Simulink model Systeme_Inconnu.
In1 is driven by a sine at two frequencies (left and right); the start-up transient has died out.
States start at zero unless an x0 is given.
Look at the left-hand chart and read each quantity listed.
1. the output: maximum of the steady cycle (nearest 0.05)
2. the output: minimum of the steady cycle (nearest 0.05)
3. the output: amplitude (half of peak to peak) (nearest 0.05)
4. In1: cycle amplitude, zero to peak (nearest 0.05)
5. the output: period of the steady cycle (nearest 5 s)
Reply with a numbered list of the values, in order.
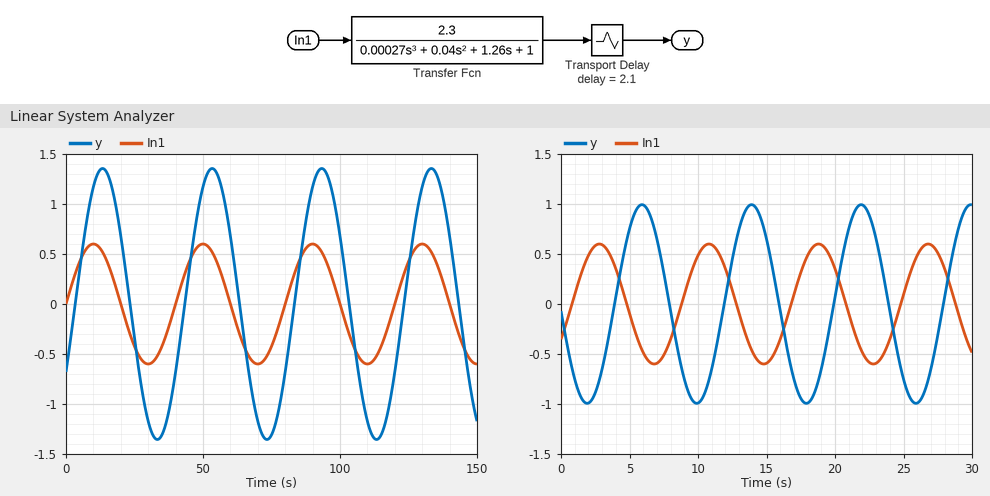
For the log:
1. 1.35
2. -1.35
3. 1.35
4. 0.60
5. 40 s
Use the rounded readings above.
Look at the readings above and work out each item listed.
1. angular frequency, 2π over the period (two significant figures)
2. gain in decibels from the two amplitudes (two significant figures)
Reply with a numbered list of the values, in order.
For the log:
1. 0.16 rad/s
2. 7.0 dB
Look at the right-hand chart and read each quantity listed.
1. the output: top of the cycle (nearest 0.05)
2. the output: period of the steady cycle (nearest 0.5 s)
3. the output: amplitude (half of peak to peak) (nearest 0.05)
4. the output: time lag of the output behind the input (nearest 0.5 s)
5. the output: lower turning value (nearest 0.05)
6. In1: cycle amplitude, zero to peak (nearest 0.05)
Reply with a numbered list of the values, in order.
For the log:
1. 1.00
2. 8.0 s
3. 1.00
4. 3.0 s
5. -1.00
6. 0.60
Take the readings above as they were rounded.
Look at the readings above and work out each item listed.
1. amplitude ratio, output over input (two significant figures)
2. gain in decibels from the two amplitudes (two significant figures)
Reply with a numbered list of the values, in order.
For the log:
1. 1.7
2. 4.4 dB
